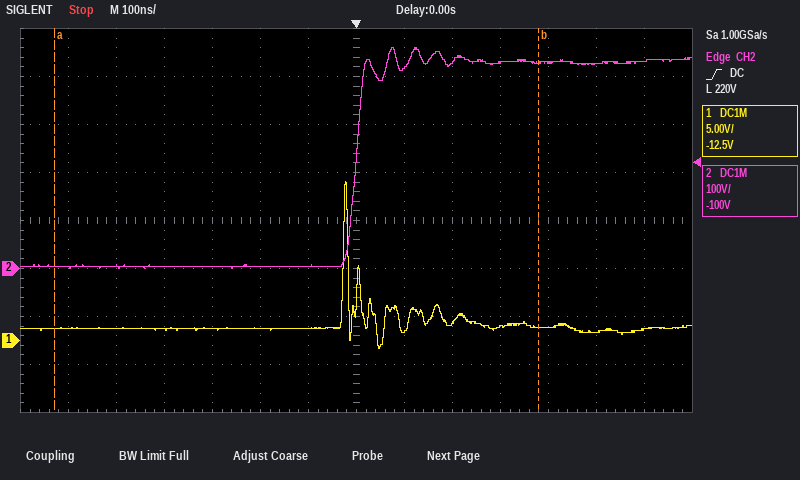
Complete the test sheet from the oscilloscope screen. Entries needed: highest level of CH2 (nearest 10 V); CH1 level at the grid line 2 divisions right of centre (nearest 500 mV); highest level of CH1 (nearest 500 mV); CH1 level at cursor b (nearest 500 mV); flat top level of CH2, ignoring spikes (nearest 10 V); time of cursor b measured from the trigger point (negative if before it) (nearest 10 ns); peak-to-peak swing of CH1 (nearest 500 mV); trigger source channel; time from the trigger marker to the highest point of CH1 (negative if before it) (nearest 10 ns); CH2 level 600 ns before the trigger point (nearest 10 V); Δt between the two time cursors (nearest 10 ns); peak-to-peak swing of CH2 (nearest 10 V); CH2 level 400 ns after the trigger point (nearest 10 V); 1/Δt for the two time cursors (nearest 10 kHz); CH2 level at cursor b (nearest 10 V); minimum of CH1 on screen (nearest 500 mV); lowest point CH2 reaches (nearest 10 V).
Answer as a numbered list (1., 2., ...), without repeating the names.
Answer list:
1. 460 V
2. 2.0 V
3. 16.5 V
4. 1.5 V
5. 430 V
6. +380 ns
7. 17.5 V
8. CH2
9. -20 ns
10. 0 V
11. 1.01 µs
12. 460 V
13. 430 V
14. 990 kHz
15. 430 V
16. -1.0 V
17. 0 V
